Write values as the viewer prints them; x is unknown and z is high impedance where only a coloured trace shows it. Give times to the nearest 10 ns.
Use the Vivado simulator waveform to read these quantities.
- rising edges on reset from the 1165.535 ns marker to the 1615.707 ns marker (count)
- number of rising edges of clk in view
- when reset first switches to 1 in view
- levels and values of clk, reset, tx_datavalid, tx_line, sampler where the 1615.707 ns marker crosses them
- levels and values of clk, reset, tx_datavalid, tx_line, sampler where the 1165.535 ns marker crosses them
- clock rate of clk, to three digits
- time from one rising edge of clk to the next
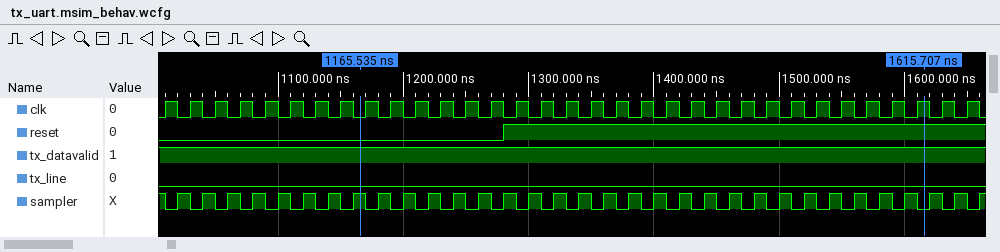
1
33
1280 ns
clk=1, reset=1, tx_datavalid=1, tx_line=0, sampler=0
clk=0, reset=0, tx_datavalid=1, tx_line=0, sampler=1
50.0 MHz
20 ns
